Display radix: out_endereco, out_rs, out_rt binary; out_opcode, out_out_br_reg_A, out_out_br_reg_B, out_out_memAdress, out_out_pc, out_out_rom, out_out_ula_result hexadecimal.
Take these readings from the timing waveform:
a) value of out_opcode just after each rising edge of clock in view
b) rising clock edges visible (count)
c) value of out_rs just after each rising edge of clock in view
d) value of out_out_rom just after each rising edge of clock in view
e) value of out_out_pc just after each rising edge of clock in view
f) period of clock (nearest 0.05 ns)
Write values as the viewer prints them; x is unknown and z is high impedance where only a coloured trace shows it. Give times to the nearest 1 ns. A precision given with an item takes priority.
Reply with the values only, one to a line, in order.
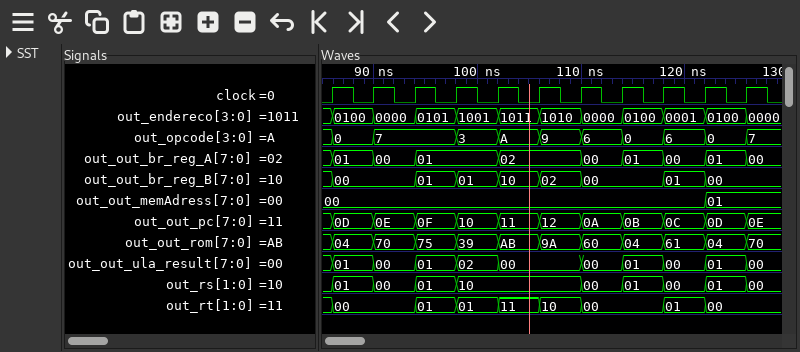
0, 7, 7, 3, A, 9, 6, 0, 6, 0, 7
11
01, 00, 01, 10, 10, 10, 00, 01, 00, 01, 00
04, 70, 75, 39, AB, 9A, 60, 04, 61, 04, 70
0D, 0E, 0F, 10, 11, 12, 0A, 0B, 0C, 0D, 0E
4 ns
